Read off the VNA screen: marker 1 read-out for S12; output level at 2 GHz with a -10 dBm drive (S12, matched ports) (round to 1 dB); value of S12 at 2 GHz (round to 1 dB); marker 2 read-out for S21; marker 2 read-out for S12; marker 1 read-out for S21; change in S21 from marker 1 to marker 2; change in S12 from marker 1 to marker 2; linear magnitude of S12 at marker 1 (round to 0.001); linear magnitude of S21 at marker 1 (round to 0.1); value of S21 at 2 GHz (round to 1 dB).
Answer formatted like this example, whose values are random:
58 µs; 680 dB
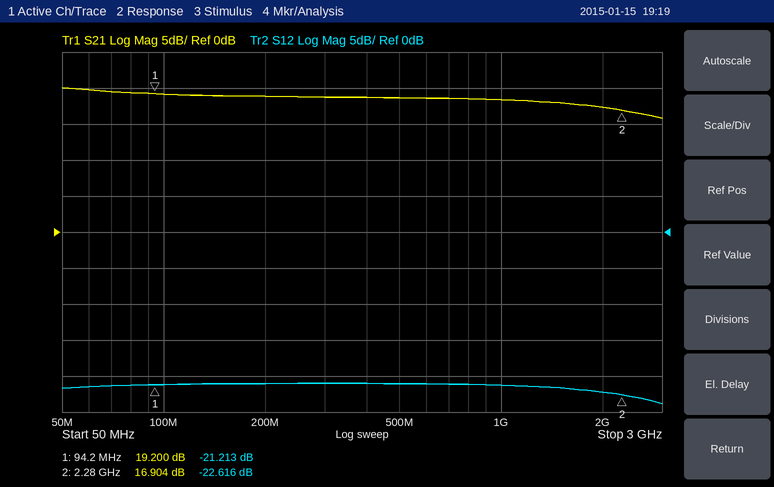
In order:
-21.213 dB; -32 dBm; -22 dB; 16.904 dB; -22.616 dB; 19.200 dB; -2.296 dB; -1.403 dB; 0.087; 9.1; 17 dB
